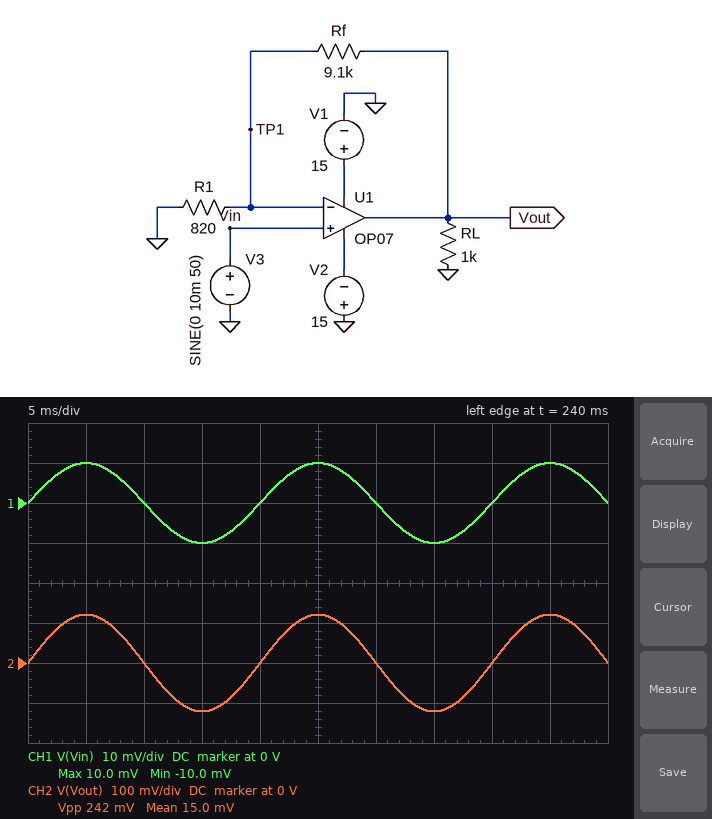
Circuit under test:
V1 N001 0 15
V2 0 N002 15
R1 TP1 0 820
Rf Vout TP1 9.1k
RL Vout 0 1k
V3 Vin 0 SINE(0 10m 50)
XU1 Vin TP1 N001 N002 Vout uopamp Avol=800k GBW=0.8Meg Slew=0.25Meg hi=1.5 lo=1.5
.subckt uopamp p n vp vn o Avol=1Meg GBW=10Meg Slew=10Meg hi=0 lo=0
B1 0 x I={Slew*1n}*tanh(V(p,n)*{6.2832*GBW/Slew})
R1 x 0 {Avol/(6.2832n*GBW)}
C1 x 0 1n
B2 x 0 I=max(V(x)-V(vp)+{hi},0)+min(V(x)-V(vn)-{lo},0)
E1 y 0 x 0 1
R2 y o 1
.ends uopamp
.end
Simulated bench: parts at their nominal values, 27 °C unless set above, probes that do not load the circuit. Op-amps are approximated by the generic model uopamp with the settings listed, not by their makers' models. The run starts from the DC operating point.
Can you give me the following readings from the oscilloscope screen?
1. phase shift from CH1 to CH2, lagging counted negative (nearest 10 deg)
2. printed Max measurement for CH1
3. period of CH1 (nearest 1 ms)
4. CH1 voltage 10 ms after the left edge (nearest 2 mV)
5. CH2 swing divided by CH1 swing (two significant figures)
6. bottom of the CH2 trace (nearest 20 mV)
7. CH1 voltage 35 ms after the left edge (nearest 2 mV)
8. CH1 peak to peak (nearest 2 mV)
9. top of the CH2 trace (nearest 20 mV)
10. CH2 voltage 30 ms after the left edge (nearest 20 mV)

0 deg
10.0 mV
20 ms
0 V
12
-120 mV
-10 mV
20 mV
120 mV
0 V
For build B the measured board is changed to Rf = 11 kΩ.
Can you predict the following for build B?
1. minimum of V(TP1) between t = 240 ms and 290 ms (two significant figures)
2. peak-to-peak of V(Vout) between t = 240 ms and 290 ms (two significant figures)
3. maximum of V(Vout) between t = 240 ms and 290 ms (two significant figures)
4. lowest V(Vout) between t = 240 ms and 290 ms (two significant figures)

-10 mV
290 mV
140 mV
-140 mV
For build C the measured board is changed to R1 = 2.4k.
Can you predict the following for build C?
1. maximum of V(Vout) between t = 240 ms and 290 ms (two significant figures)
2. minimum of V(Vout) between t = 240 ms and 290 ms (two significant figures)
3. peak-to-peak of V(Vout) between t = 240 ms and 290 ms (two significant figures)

48 mV
-48 mV
96 mV
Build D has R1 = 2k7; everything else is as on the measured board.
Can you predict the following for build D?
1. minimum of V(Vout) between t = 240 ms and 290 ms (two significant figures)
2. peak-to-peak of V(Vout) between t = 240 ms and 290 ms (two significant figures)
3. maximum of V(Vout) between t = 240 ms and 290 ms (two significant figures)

-44 mV
87 mV
44 mV
